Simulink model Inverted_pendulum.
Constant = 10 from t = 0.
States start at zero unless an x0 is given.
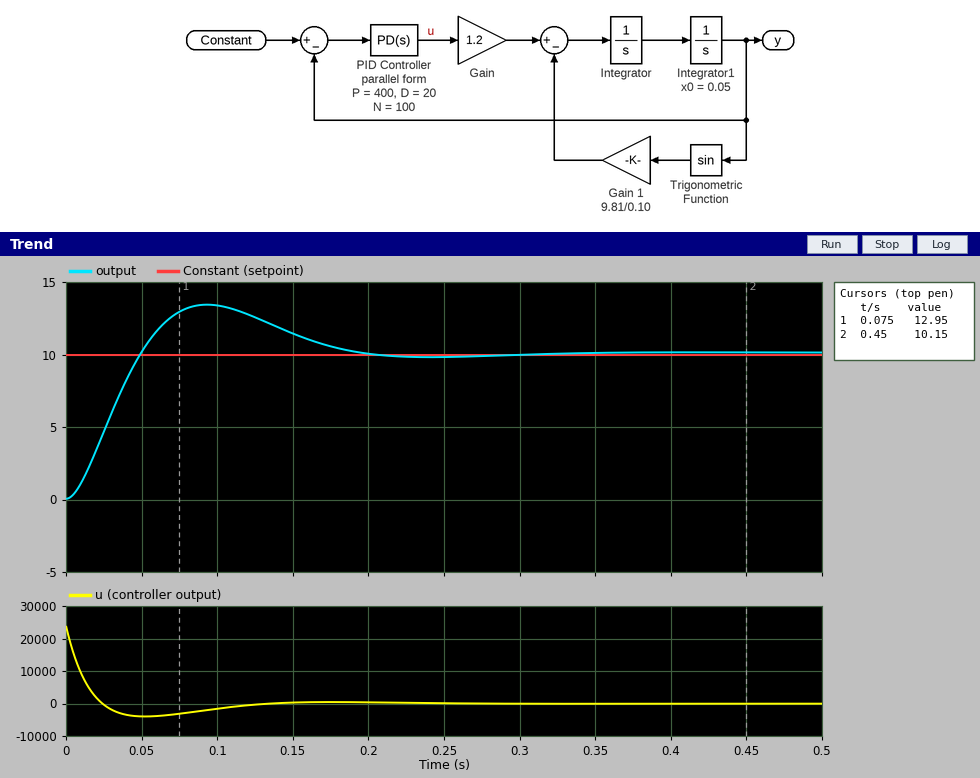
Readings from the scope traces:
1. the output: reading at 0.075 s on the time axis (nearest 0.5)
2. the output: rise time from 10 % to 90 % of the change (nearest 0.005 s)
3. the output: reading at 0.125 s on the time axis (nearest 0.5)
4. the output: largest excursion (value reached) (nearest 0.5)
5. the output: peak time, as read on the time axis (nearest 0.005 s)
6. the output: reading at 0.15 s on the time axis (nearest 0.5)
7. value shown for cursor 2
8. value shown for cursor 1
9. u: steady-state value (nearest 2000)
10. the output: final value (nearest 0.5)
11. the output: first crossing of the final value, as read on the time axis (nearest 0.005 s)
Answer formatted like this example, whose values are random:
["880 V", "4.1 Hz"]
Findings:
["13.0", "0.035 s", "12.5", "13.5", "0.095 s", "11.5", "10.15", "12.95", "0", "10.0", "0.050 s"]
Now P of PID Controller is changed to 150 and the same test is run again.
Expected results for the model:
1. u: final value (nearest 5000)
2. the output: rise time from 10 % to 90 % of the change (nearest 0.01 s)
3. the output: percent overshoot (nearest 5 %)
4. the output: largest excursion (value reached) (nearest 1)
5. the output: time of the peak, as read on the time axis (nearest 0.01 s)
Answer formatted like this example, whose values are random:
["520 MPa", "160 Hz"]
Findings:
["0", "0.05 s", "15 %", "12", "0.13 s"]
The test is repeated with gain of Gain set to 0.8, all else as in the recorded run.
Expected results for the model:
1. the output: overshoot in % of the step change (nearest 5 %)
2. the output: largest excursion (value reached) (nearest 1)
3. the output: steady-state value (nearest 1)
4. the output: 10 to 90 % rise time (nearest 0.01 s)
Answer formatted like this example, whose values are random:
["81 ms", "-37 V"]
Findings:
["35 %", "14", "10", "0.05 s"]
